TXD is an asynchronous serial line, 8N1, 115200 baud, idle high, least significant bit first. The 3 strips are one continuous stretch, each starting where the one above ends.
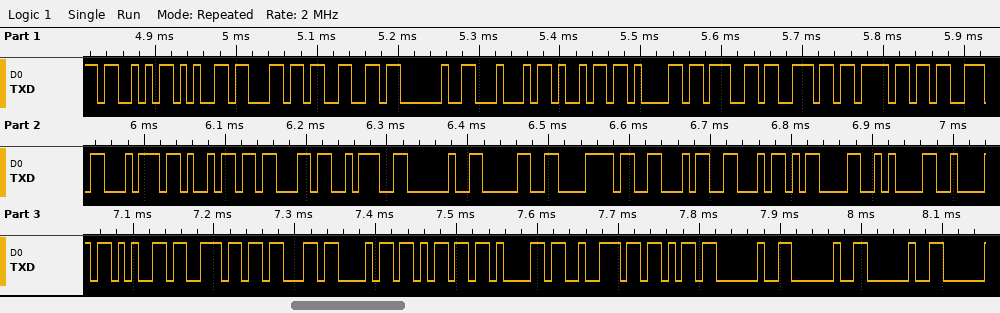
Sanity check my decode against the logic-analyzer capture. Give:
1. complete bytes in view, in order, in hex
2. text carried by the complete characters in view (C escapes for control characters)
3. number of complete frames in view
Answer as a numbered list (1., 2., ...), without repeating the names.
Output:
1. 53 65 6C 66 20 44 69 61 67 6E 6F 73 74 69 63 3A 20 30 78 46 46 0D 0A 42 65 6E 63 68 6D 61 72 6B 20 20 20
2. "Self Diagnostic: 0xFF\r\nBenchmark   "
3. 35
